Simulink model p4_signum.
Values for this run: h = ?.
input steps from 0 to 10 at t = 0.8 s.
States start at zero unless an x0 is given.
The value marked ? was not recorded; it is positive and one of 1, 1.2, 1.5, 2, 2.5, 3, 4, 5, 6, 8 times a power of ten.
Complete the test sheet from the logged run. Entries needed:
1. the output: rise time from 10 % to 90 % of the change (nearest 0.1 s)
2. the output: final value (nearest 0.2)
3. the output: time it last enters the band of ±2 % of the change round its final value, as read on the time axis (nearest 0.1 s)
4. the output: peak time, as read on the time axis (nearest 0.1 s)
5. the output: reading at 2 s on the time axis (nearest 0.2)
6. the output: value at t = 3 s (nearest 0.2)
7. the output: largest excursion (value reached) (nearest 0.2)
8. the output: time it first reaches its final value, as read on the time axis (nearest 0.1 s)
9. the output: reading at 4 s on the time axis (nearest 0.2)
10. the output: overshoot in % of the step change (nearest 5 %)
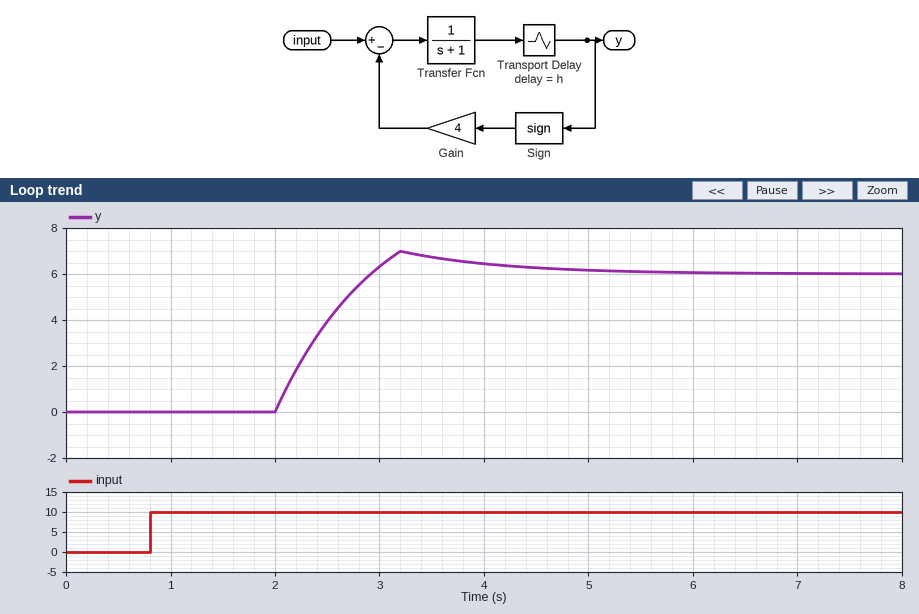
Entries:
0.7 s
6.0
5.3 s
3.2 s
0.0
6.4
7.0
2.9 s
6.4
15 %
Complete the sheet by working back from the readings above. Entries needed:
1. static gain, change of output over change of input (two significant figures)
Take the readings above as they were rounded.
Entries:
0.60
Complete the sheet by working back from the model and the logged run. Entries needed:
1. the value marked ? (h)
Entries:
1.2
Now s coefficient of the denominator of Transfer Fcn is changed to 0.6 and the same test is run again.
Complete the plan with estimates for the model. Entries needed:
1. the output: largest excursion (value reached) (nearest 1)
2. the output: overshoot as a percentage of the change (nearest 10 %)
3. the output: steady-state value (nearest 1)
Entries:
9
40 %
6
